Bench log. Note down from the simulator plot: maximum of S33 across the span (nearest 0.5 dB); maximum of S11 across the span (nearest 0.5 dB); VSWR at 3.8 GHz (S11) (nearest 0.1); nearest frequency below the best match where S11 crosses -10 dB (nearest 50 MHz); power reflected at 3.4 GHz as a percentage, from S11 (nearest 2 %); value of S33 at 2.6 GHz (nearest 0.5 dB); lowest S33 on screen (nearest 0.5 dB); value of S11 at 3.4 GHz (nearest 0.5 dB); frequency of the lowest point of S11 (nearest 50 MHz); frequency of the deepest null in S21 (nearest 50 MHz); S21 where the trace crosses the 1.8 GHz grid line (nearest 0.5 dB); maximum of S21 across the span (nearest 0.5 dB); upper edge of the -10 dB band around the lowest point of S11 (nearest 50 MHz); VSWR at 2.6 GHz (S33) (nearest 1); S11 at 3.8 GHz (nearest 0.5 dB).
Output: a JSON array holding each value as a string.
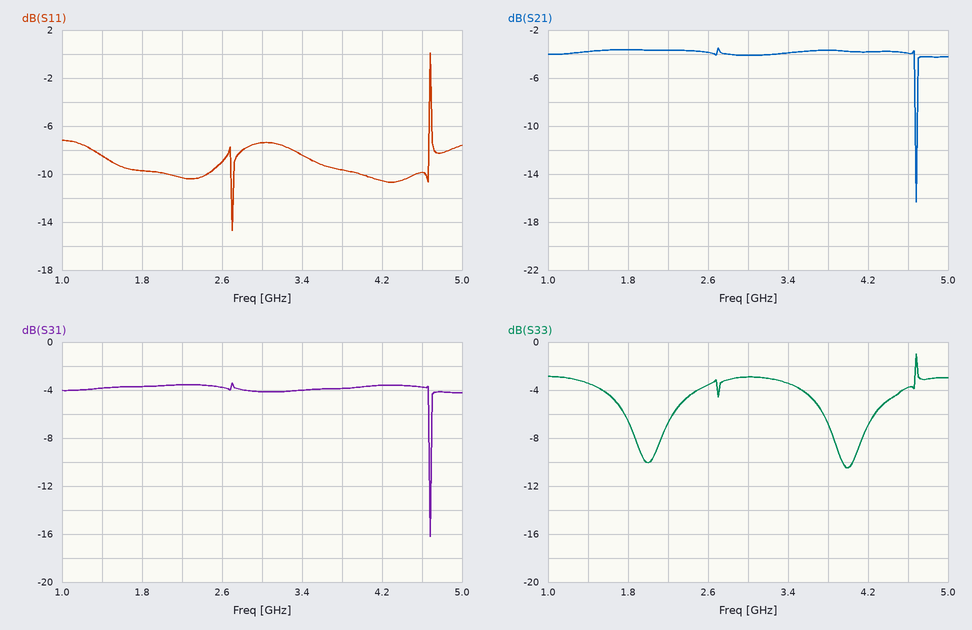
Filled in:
["-1.0 dB", "0.0 dB", "2.0", "2.70 GHz", "14 %", "-3.5 dB", "-10.5 dB", "-8.5 dB", "2.70 GHz", "4.70 GHz", "-3.5 dB", "-3.5 dB", "2.70 GHz", "5", "-9.5 dB"]
